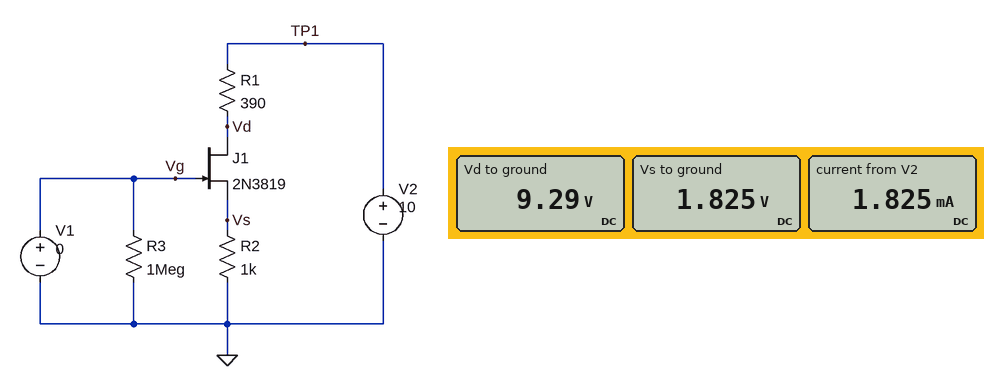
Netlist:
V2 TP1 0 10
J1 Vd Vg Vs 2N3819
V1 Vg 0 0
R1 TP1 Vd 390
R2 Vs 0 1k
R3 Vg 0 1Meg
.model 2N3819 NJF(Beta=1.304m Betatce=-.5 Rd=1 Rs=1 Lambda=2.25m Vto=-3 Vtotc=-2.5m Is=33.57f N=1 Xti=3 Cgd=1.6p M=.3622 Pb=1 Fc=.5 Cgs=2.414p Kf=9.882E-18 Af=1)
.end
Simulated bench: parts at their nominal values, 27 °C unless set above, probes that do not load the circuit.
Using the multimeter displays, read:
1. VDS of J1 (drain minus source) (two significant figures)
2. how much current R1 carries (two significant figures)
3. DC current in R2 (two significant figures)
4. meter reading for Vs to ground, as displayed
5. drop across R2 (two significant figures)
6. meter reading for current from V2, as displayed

7.5 V
1.8 mA
1.8 mA
1.825 V
1.8 V
1.825 mA
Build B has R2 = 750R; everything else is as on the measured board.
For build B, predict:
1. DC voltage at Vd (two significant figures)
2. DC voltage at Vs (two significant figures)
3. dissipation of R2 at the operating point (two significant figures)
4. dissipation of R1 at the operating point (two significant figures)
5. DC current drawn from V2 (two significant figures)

9.1 V
1.7 V
3.8 mW
2.0 mW
2.3 mA
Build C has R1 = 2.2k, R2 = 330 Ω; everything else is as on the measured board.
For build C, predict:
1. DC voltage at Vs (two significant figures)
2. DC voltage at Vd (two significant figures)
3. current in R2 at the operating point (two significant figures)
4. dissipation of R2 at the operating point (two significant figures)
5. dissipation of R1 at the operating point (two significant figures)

1.2 V
2.2 V
3.5 mA
4.1 mW
28 mW
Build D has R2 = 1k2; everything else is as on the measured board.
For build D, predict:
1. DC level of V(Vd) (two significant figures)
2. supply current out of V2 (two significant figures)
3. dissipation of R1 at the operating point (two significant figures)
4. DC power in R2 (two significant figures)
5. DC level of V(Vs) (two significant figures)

9.4 V
1.6 mA
980 µW
3.0 mW
1.9 V
